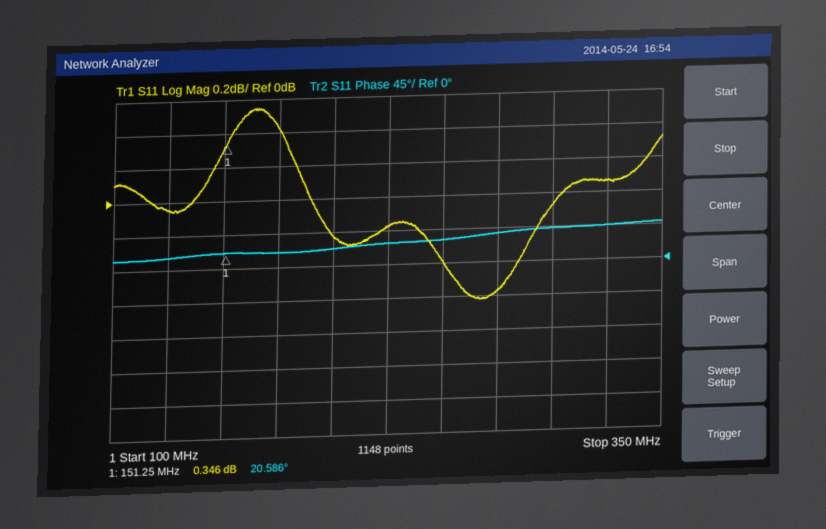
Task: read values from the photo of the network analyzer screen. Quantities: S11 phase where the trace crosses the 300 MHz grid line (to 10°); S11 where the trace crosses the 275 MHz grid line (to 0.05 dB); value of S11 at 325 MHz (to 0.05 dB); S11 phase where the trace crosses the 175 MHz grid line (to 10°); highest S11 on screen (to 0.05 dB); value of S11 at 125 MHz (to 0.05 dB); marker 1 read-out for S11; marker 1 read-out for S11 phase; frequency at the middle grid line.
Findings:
40°
-0.55 dB
0.05 dB
20°
0.55 dB
-0.05 dB
0.346 dB
20.586°
225 MHz
